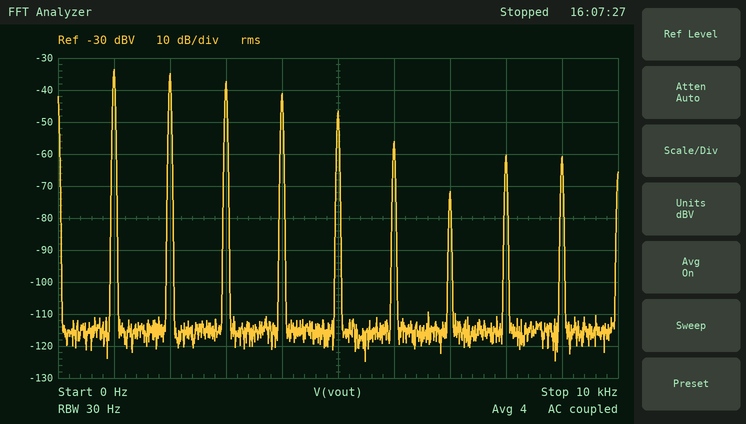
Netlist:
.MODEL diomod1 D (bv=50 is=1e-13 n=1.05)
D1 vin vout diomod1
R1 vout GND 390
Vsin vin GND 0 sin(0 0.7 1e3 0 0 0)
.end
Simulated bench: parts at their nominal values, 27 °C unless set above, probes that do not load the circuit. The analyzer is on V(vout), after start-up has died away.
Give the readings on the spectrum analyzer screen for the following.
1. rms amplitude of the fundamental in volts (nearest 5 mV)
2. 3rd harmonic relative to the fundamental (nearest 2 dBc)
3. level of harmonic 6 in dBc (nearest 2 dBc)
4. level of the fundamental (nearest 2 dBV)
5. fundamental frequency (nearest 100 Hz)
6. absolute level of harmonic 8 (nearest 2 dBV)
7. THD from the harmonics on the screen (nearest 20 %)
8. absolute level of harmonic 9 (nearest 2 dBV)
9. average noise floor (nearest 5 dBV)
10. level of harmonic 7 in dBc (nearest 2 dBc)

20 mV
-4 dBc
-22 dBc
-34 dBV
1.0 kHz
-60 dBV
120 %
-60 dBV
-115 dBV
-38 dBc
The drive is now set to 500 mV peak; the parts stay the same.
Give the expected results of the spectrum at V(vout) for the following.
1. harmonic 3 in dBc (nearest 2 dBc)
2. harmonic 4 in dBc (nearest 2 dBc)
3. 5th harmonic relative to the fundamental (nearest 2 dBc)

-2 dBc
-4 dBc
-6 dBc
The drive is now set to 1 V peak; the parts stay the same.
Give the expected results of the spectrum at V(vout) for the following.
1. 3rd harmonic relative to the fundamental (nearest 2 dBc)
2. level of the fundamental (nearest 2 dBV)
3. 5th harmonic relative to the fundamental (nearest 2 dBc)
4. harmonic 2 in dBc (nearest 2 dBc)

-8 dBc
-20 dBV
-32 dBc
-2 dBc
